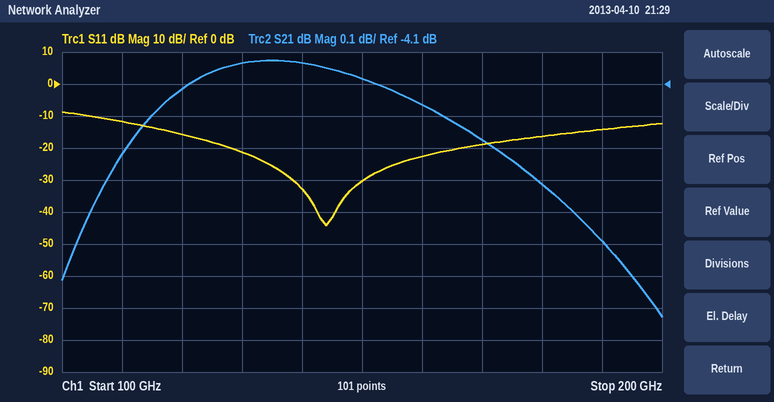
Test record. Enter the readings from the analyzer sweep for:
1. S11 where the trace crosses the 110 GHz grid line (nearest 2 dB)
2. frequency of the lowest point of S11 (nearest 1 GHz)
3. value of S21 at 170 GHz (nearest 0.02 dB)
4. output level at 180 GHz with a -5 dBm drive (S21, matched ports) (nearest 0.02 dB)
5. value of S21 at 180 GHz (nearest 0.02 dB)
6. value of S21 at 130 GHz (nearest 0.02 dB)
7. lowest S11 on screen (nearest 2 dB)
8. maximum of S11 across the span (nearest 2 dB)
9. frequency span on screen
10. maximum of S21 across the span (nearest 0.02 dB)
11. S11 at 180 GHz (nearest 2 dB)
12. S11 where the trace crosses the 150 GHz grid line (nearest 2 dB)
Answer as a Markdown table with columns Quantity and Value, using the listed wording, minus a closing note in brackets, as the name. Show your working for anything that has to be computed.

| Quantity | Value |
|---|---|
| S11 where the trace crosses the 110 GHz grid line | -12 dB |
| frequency of the lowest point of S11 | 144 GHz |
| value of S21 at 170 GHz | -4.28 dB |
| output level at 180 GHz with a -5 dBm drive (S21, matched ports) | -5 dBm + (-4.42 dB) = -9.42 dBm |
| value of S21 at 180 GHz | -4.42 dB |
| value of S21 at 130 GHz | -4.04 dB |
| lowest S11 on screen | -44 dB |
| maximum of S11 across the span | -8 dB |
| frequency span on screen | 100 GHz |
| maximum of S21 across the span | -4.02 dB |
| S11 at 180 GHz | -16 dB |
| S11 where the trace crosses the 150 GHz grid line | -30 dB |
